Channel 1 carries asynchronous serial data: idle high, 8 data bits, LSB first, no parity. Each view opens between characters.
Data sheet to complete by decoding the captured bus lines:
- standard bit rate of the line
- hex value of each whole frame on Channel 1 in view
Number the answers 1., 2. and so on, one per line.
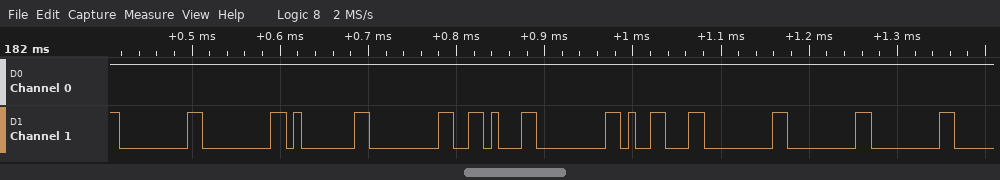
1. 115200 baud
2. 00, 00, 01, 00, 16, 00, 19, 00, 00, 00
